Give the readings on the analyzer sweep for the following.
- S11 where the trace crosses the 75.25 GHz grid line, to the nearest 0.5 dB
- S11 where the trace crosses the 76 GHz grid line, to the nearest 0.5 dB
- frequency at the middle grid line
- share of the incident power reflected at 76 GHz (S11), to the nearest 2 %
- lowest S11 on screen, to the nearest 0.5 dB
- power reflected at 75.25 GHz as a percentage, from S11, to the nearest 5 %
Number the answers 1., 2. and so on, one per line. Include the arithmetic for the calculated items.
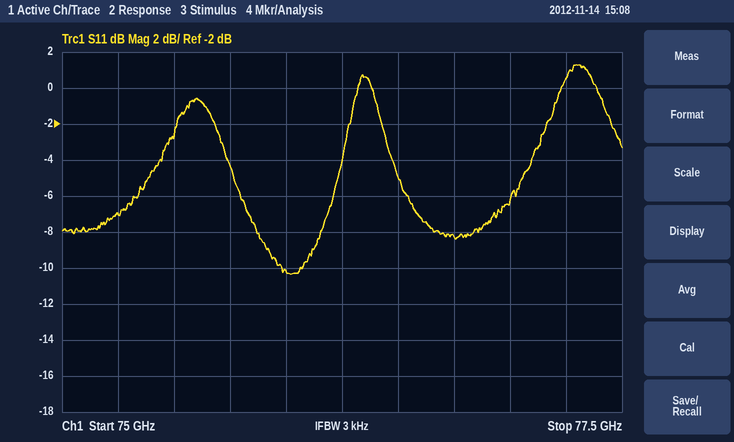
1. -7.0 dB
2. -10.0 dB
3. 76.25 GHz
4. 10^(-10/10) ≈ 10 %
5. -10.5 dB
6. 10^(-7/10) ≈ 20 %
